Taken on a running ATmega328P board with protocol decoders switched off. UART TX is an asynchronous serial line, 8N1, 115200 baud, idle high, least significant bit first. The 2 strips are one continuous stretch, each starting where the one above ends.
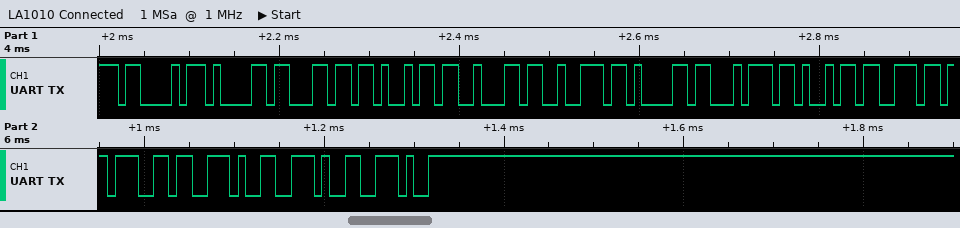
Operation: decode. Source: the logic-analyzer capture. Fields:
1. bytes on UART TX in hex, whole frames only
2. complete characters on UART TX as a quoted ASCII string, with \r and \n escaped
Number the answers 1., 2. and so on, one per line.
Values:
1. 43 61 6C 69 62 72 61 74 69 6E 67 2E 2E 2E
2. "Calibrating..."
